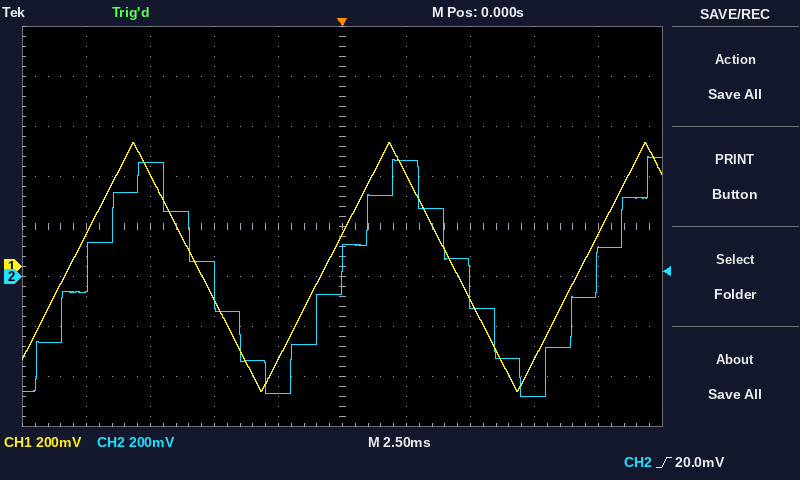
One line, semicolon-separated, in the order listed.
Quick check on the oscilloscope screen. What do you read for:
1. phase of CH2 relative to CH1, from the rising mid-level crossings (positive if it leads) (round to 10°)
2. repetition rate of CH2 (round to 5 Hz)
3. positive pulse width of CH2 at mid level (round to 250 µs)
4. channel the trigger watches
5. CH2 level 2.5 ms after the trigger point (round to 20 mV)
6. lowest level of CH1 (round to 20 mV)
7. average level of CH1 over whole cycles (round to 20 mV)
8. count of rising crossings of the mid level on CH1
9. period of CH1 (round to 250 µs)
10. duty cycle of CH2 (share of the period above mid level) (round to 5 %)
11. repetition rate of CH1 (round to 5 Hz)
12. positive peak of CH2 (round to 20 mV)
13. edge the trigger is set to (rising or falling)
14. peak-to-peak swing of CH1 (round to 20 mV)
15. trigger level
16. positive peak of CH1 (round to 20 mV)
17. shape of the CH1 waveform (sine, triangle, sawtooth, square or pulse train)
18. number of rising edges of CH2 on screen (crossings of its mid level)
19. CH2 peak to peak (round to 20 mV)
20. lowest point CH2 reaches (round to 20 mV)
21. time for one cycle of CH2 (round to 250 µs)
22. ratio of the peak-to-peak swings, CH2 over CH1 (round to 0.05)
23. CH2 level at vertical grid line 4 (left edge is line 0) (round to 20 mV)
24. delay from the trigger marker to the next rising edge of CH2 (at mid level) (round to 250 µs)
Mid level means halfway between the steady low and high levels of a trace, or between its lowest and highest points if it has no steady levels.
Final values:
-20°; 100 Hz; 5.00 ms; CH2; 460 mV; -500 mV; 0 mV; 3; 10.00 ms; 50 %; 100 Hz; 480 mV; rising; 1.00 V; 20.0 mV; 500 mV; triangle; 3; 960 mV; -480 mV; 10.00 ms; 0.95; -460 mV; 10.00 ms
